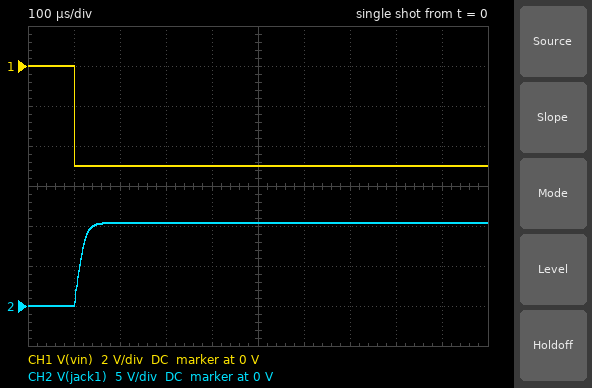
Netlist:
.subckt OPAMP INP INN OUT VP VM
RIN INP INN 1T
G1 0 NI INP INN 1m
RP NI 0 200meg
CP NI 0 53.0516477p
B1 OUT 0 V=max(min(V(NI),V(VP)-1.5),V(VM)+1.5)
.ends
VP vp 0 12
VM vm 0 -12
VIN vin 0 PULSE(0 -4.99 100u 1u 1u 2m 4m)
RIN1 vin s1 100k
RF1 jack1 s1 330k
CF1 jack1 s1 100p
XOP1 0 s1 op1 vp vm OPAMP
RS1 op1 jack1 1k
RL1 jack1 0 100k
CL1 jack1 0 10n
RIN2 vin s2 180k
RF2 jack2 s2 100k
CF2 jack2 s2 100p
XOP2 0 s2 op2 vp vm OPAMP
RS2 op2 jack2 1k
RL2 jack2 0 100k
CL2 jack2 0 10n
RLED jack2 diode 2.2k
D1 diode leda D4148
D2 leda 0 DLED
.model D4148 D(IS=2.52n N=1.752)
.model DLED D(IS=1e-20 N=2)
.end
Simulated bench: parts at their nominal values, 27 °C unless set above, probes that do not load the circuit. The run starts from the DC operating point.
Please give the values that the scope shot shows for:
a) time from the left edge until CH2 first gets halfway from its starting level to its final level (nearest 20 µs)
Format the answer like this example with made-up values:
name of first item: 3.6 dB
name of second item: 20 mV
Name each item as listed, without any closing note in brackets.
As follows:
time from the left edge until CH2 first gets halfway from its starting level to its final level: 120 µs
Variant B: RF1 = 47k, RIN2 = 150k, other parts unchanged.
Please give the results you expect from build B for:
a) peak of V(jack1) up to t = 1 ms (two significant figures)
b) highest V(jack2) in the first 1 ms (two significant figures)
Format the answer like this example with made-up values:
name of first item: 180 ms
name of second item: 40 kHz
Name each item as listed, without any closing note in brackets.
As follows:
peak of V(jack1) up to t = 1 ms: 2.4 V
highest V(jack2) in the first 1 ms: 3.3 V
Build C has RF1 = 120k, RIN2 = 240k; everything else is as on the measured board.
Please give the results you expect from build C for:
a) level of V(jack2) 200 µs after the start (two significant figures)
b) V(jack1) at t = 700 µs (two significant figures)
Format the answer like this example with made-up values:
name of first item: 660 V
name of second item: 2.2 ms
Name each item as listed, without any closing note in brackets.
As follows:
level of V(jack2) 200 µs after the start: 2.1 V
V(jack1) at t = 700 µs: 6.0 V
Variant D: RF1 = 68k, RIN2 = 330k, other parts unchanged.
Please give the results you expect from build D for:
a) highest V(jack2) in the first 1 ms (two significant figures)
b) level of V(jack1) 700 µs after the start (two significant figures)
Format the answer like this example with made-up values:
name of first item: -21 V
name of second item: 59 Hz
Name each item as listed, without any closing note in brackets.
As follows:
highest V(jack2) in the first 1 ms: 1.5 V
level of V(jack1) 700 µs after the start: 3.4 V
